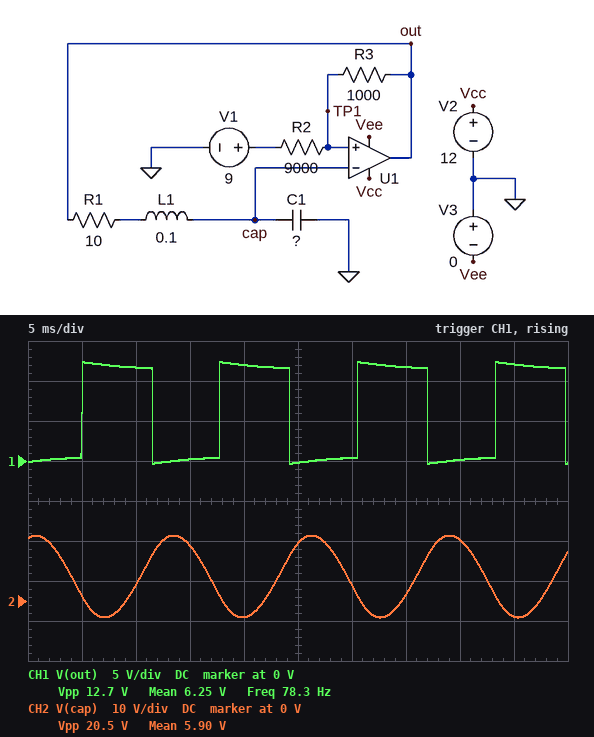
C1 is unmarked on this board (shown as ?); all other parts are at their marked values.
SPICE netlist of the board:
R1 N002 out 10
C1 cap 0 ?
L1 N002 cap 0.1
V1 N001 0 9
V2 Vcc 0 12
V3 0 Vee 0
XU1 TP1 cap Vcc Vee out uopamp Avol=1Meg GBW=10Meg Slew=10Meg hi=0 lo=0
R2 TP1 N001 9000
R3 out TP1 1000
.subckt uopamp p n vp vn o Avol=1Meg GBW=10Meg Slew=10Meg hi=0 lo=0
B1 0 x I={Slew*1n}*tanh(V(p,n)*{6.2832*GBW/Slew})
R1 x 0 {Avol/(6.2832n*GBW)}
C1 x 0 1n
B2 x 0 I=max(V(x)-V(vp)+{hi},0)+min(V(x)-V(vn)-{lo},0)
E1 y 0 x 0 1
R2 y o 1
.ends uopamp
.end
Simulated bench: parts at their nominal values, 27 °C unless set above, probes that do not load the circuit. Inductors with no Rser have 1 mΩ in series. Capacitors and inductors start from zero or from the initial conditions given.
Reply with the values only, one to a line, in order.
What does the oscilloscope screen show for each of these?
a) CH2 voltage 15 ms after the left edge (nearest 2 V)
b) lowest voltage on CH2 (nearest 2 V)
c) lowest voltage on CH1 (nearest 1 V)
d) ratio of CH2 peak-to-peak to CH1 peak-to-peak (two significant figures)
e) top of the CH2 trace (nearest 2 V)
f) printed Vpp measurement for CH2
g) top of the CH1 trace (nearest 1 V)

14 V
-4 V
0 V
1.6
16 V
20.5 V
12 V
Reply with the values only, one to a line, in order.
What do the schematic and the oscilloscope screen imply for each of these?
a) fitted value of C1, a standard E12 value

68 µF
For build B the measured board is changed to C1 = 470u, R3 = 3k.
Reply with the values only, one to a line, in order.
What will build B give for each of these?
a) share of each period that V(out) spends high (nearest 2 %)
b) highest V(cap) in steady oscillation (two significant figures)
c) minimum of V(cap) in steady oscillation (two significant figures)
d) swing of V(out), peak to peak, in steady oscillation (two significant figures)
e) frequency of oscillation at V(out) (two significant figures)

54 %
12 V
860 mV
13 V
32 Hz
